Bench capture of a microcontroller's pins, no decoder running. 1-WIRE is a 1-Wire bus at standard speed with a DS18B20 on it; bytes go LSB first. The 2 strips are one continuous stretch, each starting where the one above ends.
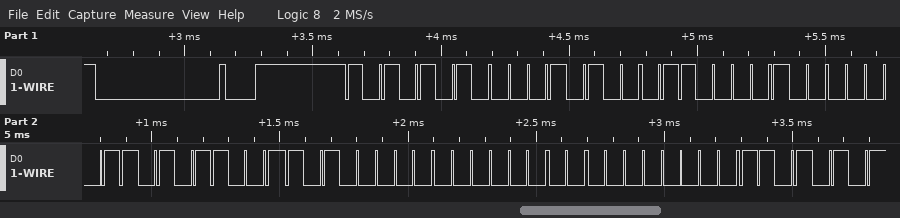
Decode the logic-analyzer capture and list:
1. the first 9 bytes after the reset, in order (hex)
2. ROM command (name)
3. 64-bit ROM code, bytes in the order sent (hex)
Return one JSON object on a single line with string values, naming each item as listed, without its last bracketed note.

{"the first 9 bytes after the reset, in order": "55 28 86 C0 9A 05 00 00 AB", "ROM command": "Match ROM", "64-bit ROM code, bytes in the order sent": "28 86 C0 9A 05 00 00 AB"}
